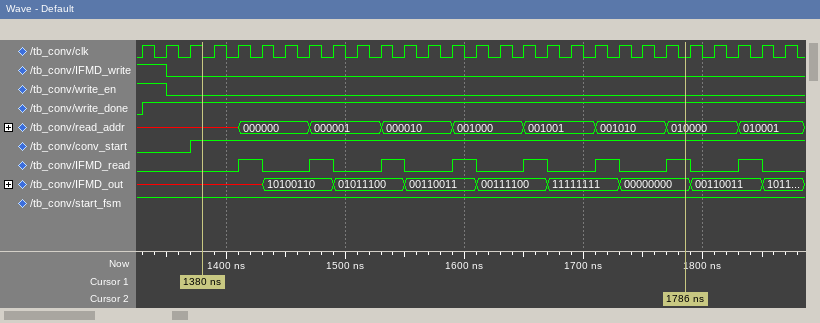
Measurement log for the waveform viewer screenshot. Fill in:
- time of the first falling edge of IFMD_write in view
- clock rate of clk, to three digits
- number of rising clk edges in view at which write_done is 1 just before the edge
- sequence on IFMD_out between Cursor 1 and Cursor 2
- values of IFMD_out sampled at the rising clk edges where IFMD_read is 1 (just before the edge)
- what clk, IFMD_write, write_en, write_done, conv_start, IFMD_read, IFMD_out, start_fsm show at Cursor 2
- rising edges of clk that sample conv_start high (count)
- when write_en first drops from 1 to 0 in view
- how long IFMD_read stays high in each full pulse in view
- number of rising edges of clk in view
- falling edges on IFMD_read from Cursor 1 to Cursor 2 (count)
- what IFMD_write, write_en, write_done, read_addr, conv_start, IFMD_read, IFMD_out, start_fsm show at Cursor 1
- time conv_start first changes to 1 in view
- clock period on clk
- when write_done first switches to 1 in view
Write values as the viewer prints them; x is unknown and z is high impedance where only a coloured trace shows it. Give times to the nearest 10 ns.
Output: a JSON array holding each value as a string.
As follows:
["1350 ns", "50.0 MHz", "27", "x, 10100110, 01011100, 00110011, 00111100, 11111111, 00000000", "x, 10100110, 01011100, 00110011, 00111100, 11111111, 00000000, 00110011", "clk=0, IFMD_write=0, write_en=0, write_done=1, conv_start=1, IFMD_read=1, IFMD_out=00000000, start_fsm=1", "25", "1350 ns", "20 ns, 20 ns, 20 ns, 20 ns, 20 ns, 20 ns, 20 ns, 20 ns", "28", "6", "IFMD_write=0, write_en=0, write_done=1, read_addr=x, conv_start=1, IFMD_read=0, IFMD_out=x, start_fsm=1", "1370 ns", "20 ns", "1330 ns"]
